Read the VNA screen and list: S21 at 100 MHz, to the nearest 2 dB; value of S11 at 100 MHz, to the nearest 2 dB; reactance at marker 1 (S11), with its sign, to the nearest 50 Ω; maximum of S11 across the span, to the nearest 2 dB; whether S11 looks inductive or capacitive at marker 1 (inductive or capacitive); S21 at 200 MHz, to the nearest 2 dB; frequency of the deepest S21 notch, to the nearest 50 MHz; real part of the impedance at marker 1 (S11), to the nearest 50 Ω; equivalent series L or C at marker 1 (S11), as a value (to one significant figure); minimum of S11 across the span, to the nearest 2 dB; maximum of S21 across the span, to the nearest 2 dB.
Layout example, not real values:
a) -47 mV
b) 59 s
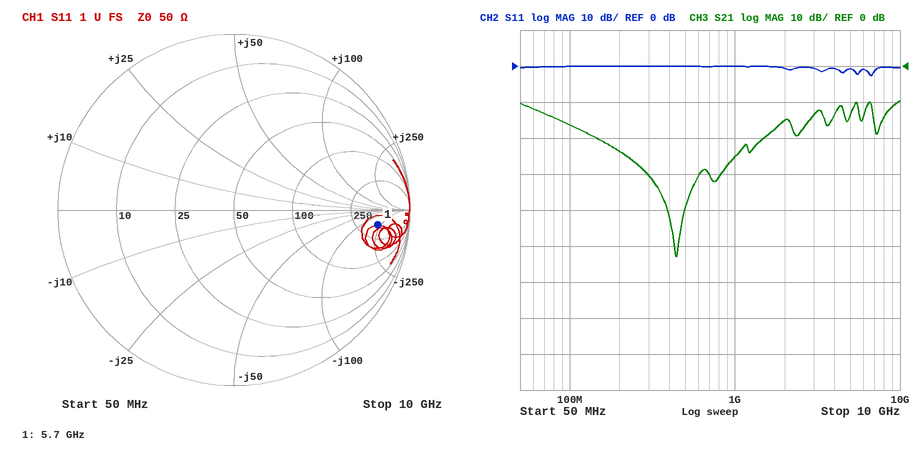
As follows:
a) -16 dB
b) 0 dB
c) -200 Ω
d) 0 dB
e) capacitive
f) -24 dB
g) 450 MHz
h) 400 Ω
i) 100 fF
j) -2 dB
k) -10 dB
